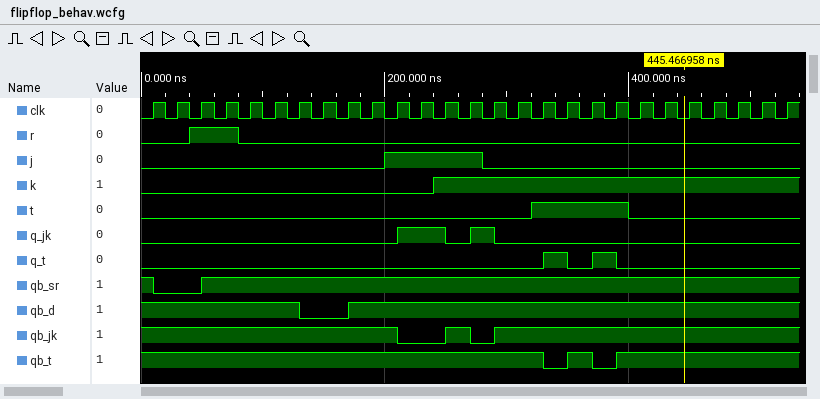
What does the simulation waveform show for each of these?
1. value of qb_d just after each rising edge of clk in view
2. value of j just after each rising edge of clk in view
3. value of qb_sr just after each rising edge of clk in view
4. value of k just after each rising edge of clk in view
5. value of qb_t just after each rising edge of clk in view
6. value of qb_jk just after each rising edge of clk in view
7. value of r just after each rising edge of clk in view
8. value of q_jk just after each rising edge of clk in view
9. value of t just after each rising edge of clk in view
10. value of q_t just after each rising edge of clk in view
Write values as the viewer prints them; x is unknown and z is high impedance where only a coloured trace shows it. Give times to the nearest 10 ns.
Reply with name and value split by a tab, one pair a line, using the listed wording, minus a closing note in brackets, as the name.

value of qb_d just after each rising edge of clk in view	1 1 1 1 1 1 0 0 1 1 1 1 1 1 1 1 1 1 1 1 1 1 1 1 1 1 1
value of j just after each rising edge of clk in view	0 0 0 0 0 0 0 0 0 0 1 1 1 1 0 0 0 0 0 0 0 0 0 0 0 0 0
value of qb_sr just after each rising edge of clk in view	0 0 1 1 1 1 1 1 1 1 1 1 1 1 1 1 1 1 1 1 1 1 1 1 1 1 1
value of k just after each rising edge of clk in view	0 0 0 0 0 0 0 0 0 0 0 0 1 1 1 1 1 1 1 1 1 1 1 1 1 1 1
value of qb_t just after each rising edge of clk in view	1 1 1 1 1 1 1 1 1 1 1 1 1 1 1 1 0 1 0 1 1 1 1 1 1 1 1
value of qb_jk just after each rising edge of clk in view	1 1 1 1 1 1 1 1 1 1 0 0 1 0 1 1 1 1 1 1 1 1 1 1 1 1 1
value of r just after each rising edge of clk in view	0 0 1 1 0 0 0 0 0 0 0 0 0 0 0 0 0 0 0 0 0 0 0 0 0 0 0
value of q_jk just after each rising edge of clk in view	0 0 0 0 0 0 0 0 0 0 1 1 0 1 0 0 0 0 0 0 0 0 0 0 0 0 0
value of t just after each rising edge of clk in view	0 0 0 0 0 0 0 0 0 0 0 0 0 0 0 0 1 1 1 1 0 0 0 0 0 0 0
value of q_t just after each rising edge of clk in view	0 0 0 0 0 0 0 0 0 0 0 0 0 0 0 0 1 0 1 0 0 0 0 0 0 0 0
